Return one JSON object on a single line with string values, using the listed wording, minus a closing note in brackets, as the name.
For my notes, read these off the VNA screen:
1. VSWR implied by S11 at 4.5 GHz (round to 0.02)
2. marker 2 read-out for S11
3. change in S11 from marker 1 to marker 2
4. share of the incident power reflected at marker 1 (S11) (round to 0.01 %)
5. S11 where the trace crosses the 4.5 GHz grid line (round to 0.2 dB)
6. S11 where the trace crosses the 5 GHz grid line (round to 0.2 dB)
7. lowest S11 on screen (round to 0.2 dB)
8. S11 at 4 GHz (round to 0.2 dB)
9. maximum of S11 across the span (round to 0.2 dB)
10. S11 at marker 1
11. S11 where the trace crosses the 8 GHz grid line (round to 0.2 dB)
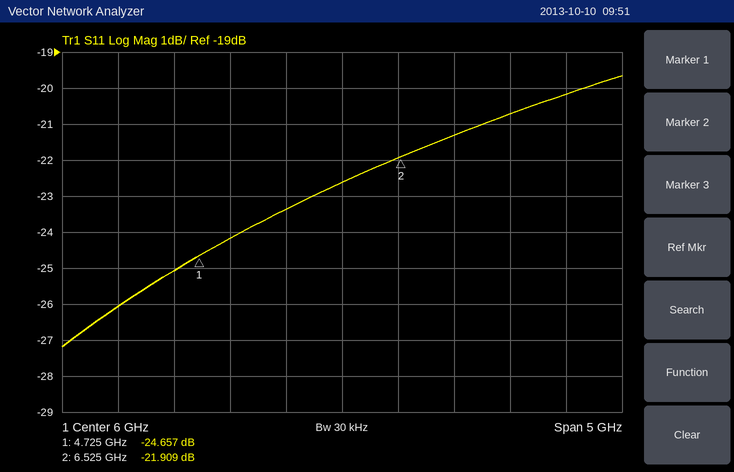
{"VSWR implied by S11 at 4.5 GHz": "1.12", "marker 2 read-out for S11": "-21.909 dB", "change in S11 from marker 1 to marker 2": "2.748 dB", "share of the incident power reflected at marker 1 (S11)": "0.34 %", "S11 where the trace crosses the 4.5 GHz grid line": "-25.0 dB", "S11 where the trace crosses the 5 GHz grid line": "-24.2 dB", "lowest S11 on screen": "-27.2 dB", "S11 at 4 GHz": "-26.0 dB", "maximum of S11 across the span": "-19.6 dB", "S11 at marker 1": "-24.657 dB", "S11 where the trace crosses the 8 GHz grid line": "-20.2 dB"}
